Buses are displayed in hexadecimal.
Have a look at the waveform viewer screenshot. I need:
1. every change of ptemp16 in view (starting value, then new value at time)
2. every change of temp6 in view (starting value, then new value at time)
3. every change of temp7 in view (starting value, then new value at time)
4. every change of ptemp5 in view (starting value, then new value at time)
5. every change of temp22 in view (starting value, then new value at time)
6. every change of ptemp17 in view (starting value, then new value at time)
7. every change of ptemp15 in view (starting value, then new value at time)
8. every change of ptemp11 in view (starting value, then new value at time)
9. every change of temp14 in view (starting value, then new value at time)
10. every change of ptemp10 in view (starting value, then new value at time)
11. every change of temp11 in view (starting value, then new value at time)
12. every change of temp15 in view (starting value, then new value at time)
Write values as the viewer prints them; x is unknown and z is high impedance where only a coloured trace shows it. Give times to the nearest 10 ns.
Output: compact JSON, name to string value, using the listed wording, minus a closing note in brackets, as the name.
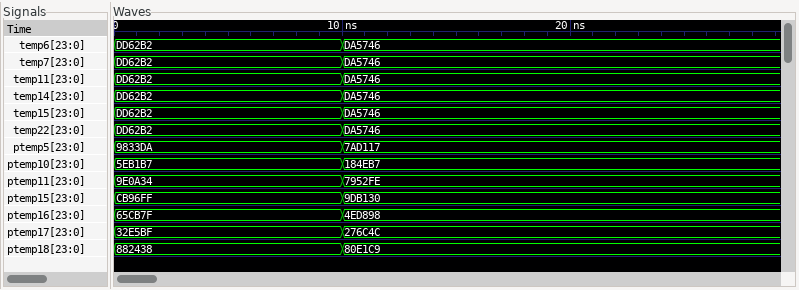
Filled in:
{"every change of ptemp16 in view": "65CB7F, 4ED898 at 10 ns", "every change of temp6 in view": "DD62B2, DA5746 at 10 ns", "every change of temp7 in view": "DD62B2, DA5746 at 10 ns", "every change of ptemp5 in view": "9833DA, 7AD117 at 10 ns", "every change of temp22 in view": "DD62B2, DA5746 at 10 ns", "every change of ptemp17 in view": "32E5BF, 276C4C at 10 ns", "every change of ptemp15 in view": "CB96FF, 9DB130 at 10 ns", "every change of ptemp11 in view": "9E0A34, 7952FE at 10 ns", "every change of temp14 in view": "DD62B2, DA5746 at 10 ns", "every change of ptemp10 in view": "5EB1B7, 184EB7 at 10 ns", "every change of temp11 in view": "DD62B2, DA5746 at 10 ns", "every change of temp15 in view": "DD62B2, DA5746 at 10 ns"}
